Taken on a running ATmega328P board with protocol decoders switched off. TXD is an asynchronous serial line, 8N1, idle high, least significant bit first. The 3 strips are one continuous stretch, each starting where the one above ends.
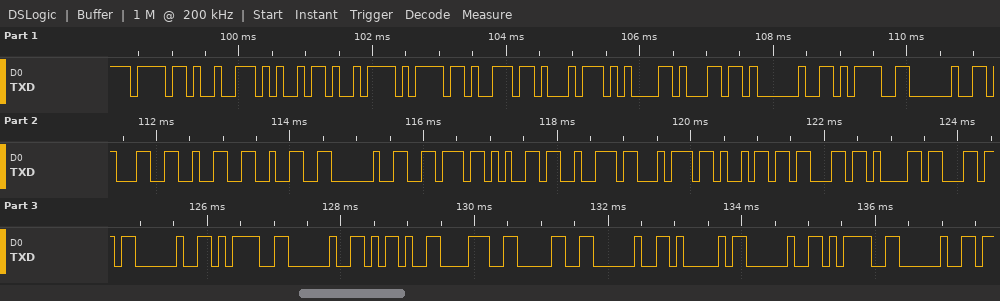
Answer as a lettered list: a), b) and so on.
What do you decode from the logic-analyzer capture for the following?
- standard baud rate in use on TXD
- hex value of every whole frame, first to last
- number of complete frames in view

a) 9600 baud
b) 6F 72 69 7A 6F 6E 74 61 6C 20 3D 20 31 32 32 20 76 65 72 74 69 63 61 6C 20 3D 20 2D 38 30 20 41 20 3D 20
c) 35
